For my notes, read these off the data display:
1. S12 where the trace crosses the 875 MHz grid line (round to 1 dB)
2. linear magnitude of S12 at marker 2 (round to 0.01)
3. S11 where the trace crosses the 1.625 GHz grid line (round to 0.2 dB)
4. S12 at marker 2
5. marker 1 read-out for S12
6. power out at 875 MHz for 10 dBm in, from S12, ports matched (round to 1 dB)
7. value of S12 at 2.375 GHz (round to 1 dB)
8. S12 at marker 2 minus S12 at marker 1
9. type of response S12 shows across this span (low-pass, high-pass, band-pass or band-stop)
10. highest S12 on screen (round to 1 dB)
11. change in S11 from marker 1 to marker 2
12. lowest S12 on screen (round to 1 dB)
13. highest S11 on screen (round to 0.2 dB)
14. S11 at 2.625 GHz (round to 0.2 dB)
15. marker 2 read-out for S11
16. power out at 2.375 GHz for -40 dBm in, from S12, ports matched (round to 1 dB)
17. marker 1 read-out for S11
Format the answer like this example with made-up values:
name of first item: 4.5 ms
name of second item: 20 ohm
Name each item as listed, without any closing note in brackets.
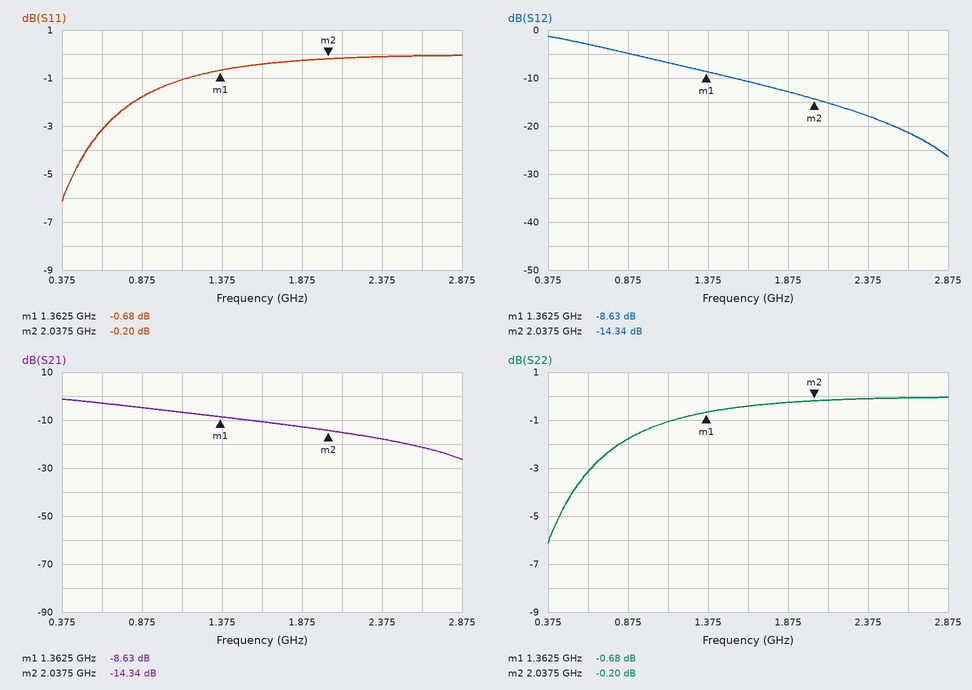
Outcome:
S12 where the trace crosses the 875 MHz grid line: -5 dB
linear magnitude of S12 at marker 2: 0.19
S11 where the trace crosses the 1.625 GHz grid line: -0.4 dB
S12 at marker 2: -14.34 dB
marker 1 read-out for S12: -8.63 dB
power out at 875 MHz for 10 dBm in, from S12, ports matched: 5 dBm
value of S12 at 2.375 GHz: -18 dB
S12 at marker 2 minus S12 at marker 1: -5.71 dB
type of response S12 shows across this span: low-pass
highest S12 on screen: -1 dB
change in S11 from marker 1 to marker 2: 0.48 dB
lowest S12 on screen: -26 dB
highest S11 on screen: 0.0 dB
S11 at 2.625 GHz: 0.0 dB
marker 2 read-out for S11: -0.20 dB
power out at 2.375 GHz for -40 dBm in, from S12, ports matched: -58 dBm
marker 1 read-out for S11: -0.68 dB
